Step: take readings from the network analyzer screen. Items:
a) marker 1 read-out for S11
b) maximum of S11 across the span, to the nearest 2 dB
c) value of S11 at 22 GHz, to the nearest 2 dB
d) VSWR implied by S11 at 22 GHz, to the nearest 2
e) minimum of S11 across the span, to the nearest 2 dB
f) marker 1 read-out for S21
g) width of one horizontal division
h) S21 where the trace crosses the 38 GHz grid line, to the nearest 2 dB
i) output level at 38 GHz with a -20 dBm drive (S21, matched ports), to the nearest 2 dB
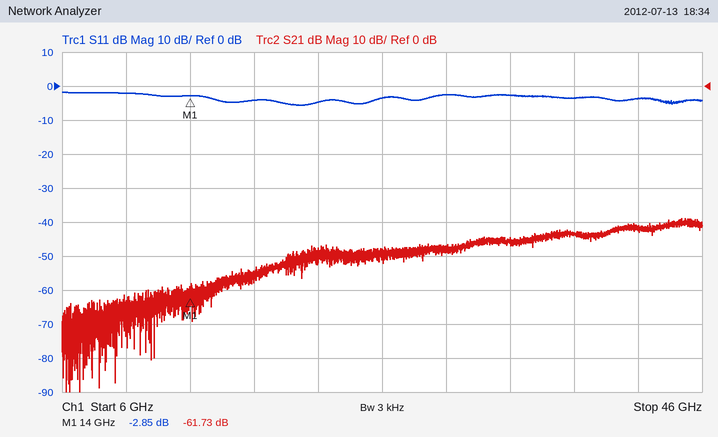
-2.85 dB
-2 dB
-4 dB
4
-6 dB
-61.73 dB
4 GHz
-44 dB
-64 dBm
